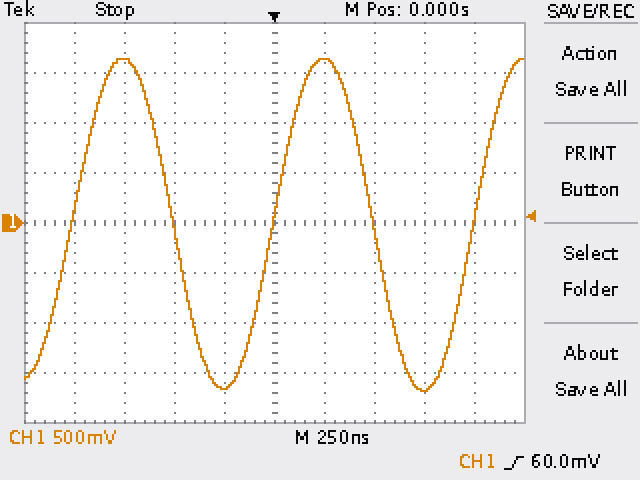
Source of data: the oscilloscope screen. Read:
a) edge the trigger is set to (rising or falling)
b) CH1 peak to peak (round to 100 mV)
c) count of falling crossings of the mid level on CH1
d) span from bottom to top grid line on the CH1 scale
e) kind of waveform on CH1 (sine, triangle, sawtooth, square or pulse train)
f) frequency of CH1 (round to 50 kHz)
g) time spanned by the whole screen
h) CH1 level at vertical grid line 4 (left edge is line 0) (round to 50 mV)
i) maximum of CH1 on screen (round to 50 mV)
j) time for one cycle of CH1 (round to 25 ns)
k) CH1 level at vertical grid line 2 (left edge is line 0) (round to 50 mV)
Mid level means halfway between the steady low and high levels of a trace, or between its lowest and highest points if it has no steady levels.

rising
3.30 V
2
4 V
sine
1.00 MHz
2.5 µs
-1.65 V
1.65 V
1.000 µs
1.65 V
